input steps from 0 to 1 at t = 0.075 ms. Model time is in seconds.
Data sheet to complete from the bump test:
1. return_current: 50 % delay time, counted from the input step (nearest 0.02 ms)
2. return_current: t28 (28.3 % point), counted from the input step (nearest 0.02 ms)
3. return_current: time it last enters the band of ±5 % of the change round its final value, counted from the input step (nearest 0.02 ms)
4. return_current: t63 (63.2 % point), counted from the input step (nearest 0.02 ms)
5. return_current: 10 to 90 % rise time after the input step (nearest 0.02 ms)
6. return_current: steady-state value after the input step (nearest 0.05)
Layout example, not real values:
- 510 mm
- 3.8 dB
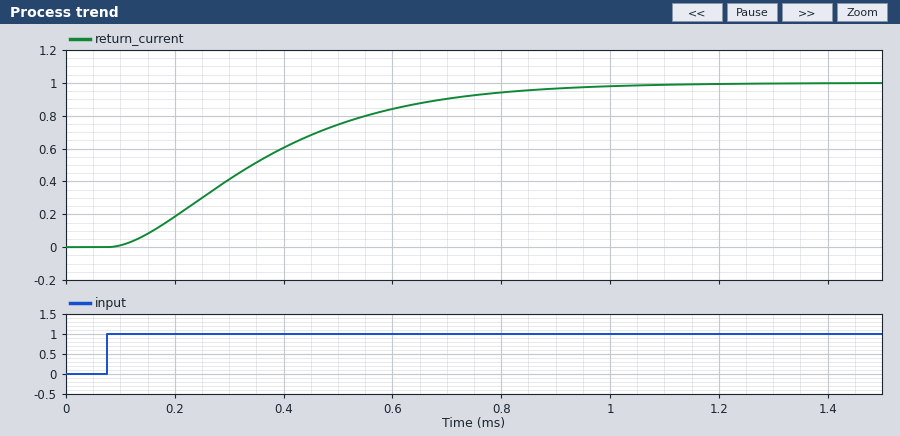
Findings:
- 0.26 ms
- 0.16 ms
- 0.76 ms
- 0.34 ms
- 0.54 ms
- 1.00
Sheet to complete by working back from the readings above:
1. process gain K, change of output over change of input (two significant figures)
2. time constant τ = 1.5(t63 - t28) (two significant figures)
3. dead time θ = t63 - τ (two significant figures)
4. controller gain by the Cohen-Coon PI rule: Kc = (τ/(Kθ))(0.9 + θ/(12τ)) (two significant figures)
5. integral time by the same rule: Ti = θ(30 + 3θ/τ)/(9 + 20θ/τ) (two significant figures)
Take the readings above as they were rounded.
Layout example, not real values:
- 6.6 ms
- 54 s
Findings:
- 1.0
- 0.27 ms
- 0.070 ms
- 3.6
- 0.15 ms
